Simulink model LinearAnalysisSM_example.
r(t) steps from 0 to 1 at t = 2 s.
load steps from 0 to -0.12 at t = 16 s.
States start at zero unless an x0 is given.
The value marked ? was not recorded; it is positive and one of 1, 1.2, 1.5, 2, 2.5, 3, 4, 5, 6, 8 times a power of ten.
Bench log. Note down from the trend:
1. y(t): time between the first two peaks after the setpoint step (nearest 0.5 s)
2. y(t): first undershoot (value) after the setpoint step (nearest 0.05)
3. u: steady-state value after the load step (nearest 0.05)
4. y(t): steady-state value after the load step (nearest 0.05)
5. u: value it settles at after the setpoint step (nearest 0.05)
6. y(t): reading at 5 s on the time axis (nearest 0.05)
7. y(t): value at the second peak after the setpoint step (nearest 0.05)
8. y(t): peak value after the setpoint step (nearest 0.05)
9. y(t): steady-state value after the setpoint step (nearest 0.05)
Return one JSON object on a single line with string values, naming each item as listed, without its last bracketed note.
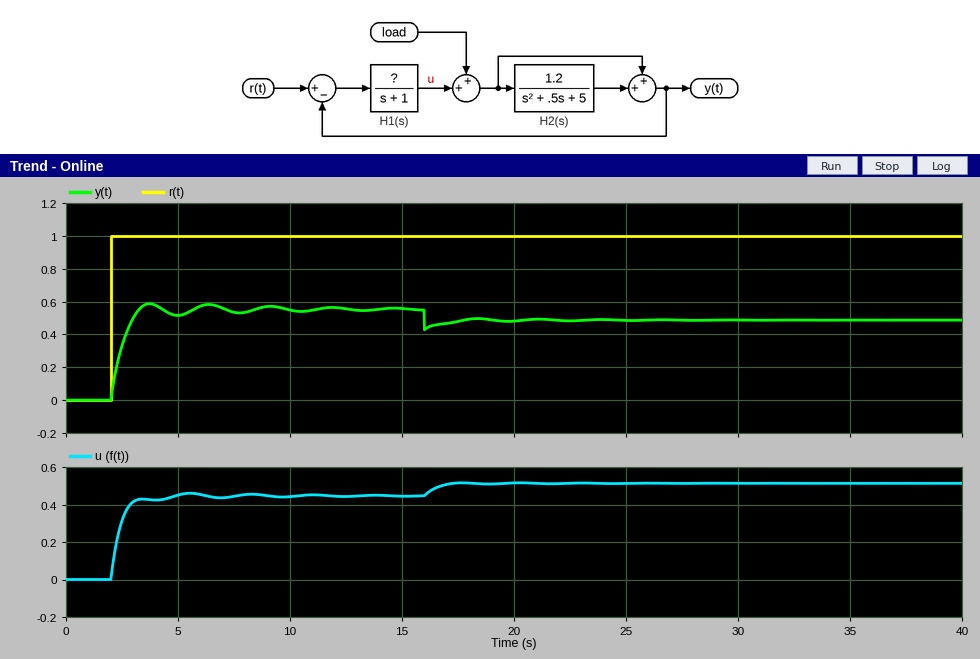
{"y(t): time between the first two peaks after the setpoint step": "2.5 s", "y(t): first undershoot (value) after the setpoint step": "0.50", "u: steady-state value after the load step": "0.50", "y(t): steady-state value after the load step": "0.50", "u: value it settles at after the setpoint step": "0.45", "y(t): reading at 5 s on the time axis": "0.50", "y(t): value at the second peak after the setpoint step": "0.60", "y(t): peak value after the setpoint step": "0.60", "y(t): steady-state value after the setpoint step": "0.55"}
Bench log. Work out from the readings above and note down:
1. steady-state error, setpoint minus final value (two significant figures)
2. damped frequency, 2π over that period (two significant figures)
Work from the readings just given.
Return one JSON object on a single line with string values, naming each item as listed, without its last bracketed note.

{"steady-state error, setpoint minus final value": "0.45", "damped frequency, 2π over that period": "2.5 rad/s"}
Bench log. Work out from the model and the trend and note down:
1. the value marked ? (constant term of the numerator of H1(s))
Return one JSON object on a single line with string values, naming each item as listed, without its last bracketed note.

{"the value marked ? (constant term of the numerator of H1(s))": "1"}
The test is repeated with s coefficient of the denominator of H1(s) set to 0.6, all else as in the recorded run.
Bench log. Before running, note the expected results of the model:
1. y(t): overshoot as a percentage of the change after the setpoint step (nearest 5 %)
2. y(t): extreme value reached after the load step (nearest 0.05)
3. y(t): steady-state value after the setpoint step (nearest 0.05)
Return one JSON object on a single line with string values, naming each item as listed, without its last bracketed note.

{"y(t): overshoot as a percentage of the change after the setpoint step": "10 %", "y(t): extreme value reached after the load step": "0.45", "y(t): steady-state value after the setpoint step": "0.55"}
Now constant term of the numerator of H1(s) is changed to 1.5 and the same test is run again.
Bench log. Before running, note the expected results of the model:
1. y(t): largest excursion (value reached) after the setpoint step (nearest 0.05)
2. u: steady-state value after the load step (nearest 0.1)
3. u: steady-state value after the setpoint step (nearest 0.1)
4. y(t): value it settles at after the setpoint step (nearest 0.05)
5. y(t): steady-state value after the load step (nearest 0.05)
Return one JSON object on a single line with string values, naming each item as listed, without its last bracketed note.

{"y(t): largest excursion (value reached) after the setpoint step": "0.70", "u: steady-state value after the load step": "0.6", "u: steady-state value after the setpoint step": "0.5", "y(t): value it settles at after the setpoint step": "0.65", "y(t): steady-state value after the load step": "0.60"}
